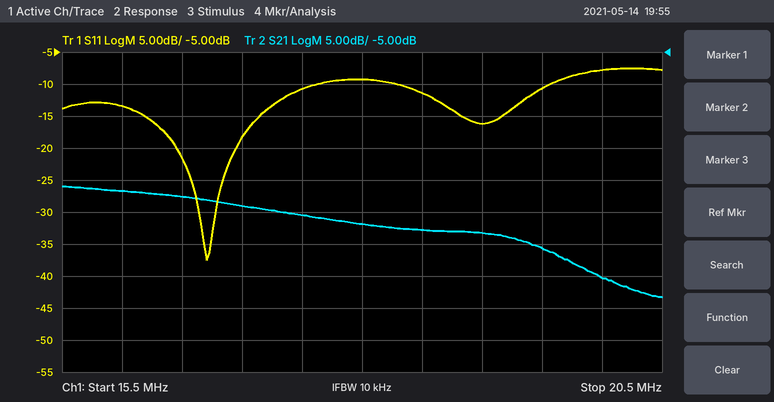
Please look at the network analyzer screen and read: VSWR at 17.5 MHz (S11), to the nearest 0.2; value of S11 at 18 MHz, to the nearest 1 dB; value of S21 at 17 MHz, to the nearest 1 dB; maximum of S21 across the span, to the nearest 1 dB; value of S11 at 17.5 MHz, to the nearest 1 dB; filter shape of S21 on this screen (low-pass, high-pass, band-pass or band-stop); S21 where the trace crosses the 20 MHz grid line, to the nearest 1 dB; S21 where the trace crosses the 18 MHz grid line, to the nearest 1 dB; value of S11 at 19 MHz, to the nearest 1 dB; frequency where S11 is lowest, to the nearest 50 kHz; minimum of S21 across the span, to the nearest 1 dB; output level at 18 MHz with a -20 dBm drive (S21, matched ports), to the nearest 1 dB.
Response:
1.8
-9 dB
-29 dB
-26 dB
-11 dB
low-pass
-40 dB
-32 dB
-16 dB
16.70 MHz
-43 dB
-52 dBm
